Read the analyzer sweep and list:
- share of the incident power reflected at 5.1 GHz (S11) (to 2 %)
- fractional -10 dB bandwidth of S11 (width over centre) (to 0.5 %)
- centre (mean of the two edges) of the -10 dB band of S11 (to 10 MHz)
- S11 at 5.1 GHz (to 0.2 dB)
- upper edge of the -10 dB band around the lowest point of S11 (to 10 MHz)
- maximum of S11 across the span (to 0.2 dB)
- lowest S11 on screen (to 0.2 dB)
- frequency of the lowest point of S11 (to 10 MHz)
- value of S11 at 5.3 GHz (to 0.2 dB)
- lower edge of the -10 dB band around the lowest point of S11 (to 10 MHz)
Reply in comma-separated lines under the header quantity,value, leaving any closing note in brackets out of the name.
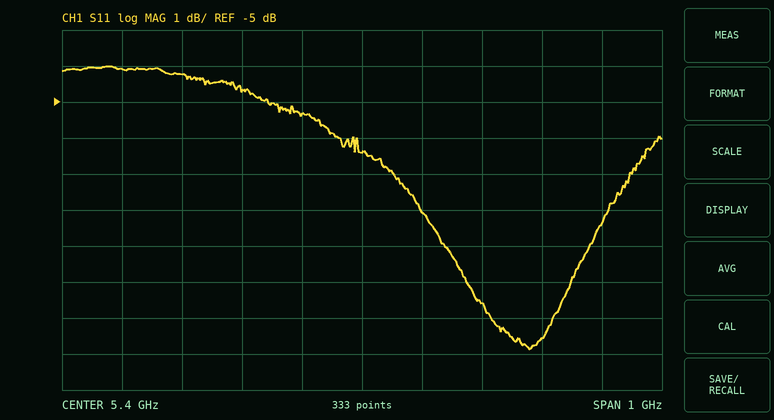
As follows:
quantity,value
share of the incident power reflected at 5.1 GHz (S11),38 %
fractional -10 dB bandwidth of S11 (width over centre),3.0 %
centre (mean of the two edges) of the -10 dB band of S11,5.66 GHz
S11 at 5.1 GHz,-4.2 dB
upper edge of the -10 dB band around the lowest point of S11,5.75 GHz
maximum of S11 across the span,-4.0 dB
lowest S11 on screen,-11.8 dB
frequency of the lowest point of S11,5.68 GHz
value of S11 at 5.3 GHz,-5.4 dB
lower edge of the -10 dB band around the lowest point of S11,5.57 GHz
